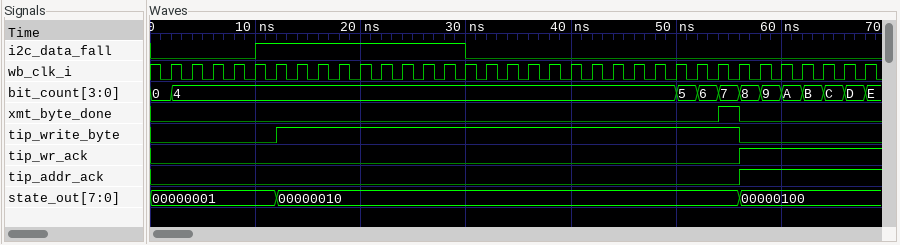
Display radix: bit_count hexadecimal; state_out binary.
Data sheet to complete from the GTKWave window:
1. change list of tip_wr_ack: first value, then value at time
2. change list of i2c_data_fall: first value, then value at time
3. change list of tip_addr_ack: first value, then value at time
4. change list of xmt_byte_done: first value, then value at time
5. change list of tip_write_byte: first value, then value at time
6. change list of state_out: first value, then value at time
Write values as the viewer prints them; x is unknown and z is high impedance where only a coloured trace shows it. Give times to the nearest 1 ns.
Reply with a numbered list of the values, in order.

1. 0, 1 at 56 ns
2. 0, 1 at 10 ns, 0 at 30 ns
3. 0, 1 at 56 ns
4. 0, 1 at 54 ns, 0 at 56 ns
5. 0, 1 at 12 ns, 0 at 56 ns
6. 00000001, 00000010 at 12 ns, 00000100 at 56 ns
